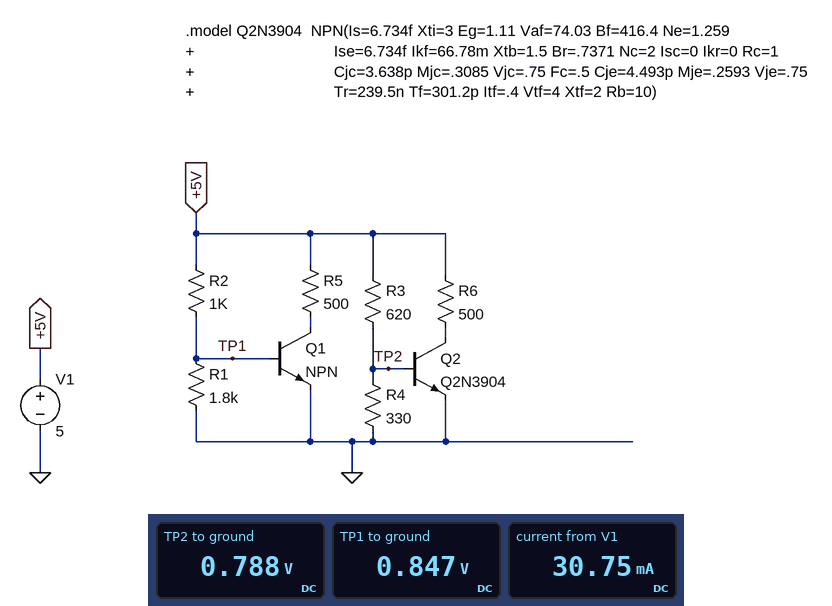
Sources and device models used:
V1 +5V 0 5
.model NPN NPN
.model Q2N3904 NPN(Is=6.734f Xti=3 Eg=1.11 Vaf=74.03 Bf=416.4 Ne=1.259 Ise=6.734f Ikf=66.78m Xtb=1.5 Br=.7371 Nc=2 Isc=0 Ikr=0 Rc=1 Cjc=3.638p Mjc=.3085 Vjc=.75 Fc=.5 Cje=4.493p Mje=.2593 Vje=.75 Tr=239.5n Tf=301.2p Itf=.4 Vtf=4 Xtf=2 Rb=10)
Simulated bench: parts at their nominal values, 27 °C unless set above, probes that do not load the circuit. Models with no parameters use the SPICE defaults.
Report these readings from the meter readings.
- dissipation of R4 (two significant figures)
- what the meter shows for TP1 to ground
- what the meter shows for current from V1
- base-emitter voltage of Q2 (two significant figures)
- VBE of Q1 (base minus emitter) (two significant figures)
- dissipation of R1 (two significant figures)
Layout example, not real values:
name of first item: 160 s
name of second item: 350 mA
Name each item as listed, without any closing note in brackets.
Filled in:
dissipation of R4: 1.9 mW
what the meter shows for TP1 to ground: 0.847 V
what the meter shows for current from V1: 30.75 mA
base-emitter voltage of Q2: 790 mV
VBE of Q1 (base minus emitter): 850 mV
dissipation of R1: 400 µW
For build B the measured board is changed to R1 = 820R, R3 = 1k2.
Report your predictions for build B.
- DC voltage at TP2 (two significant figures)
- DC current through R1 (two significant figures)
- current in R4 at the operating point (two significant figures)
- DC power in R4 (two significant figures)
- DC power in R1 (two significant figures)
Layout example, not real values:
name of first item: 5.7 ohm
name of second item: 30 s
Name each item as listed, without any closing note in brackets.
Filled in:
DC voltage at TP2: 750 mV
DC current through R1: 1.0 mA
current in R4 at the operating point: 2.3 mA
DC power in R4: 1.7 mW
DC power in R1: 870 µW
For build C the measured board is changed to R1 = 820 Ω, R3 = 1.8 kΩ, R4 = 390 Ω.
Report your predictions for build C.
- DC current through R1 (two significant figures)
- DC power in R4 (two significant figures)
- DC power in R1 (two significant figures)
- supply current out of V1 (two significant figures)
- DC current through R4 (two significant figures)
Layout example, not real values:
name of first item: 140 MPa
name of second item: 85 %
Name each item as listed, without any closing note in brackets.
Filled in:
DC current through R1: 1.0 mA
DC power in R4: 1.4 mW
DC power in R1: 870 µW
supply current out of V1: 26 mA
DC current through R4: 1.9 mA
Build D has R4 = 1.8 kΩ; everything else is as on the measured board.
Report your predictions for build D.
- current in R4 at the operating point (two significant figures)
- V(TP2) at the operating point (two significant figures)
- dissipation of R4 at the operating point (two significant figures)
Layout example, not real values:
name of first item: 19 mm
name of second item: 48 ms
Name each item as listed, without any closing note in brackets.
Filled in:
current in R4 at the operating point: 450 µA
V(TP2) at the operating point: 810 mV
dissipation of R4 at the operating point: 370 µW
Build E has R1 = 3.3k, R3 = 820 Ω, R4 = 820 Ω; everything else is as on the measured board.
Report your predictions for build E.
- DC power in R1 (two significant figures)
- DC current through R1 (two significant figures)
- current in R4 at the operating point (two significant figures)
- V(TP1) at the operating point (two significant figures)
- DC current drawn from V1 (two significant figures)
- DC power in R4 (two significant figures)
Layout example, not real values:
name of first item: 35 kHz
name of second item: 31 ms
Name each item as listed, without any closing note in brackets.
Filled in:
DC power in R1: 220 µW
DC current through R1: 260 µA
current in R4 at the operating point: 960 µA
V(TP1) at the operating point: 850 mV
DC current drawn from V1: 29 mA
DC power in R4: 750 µW
